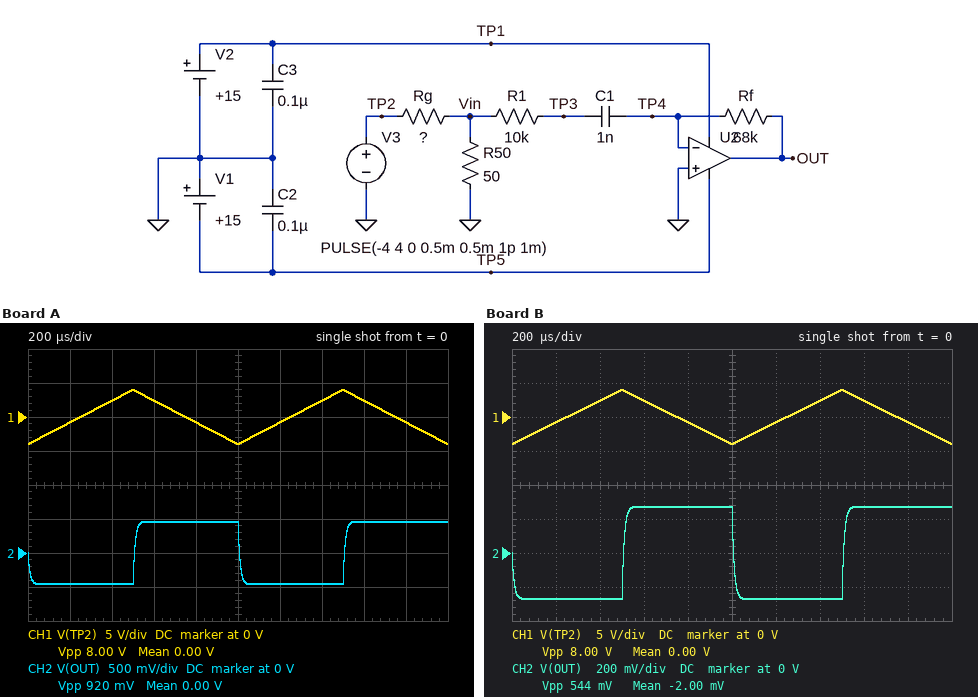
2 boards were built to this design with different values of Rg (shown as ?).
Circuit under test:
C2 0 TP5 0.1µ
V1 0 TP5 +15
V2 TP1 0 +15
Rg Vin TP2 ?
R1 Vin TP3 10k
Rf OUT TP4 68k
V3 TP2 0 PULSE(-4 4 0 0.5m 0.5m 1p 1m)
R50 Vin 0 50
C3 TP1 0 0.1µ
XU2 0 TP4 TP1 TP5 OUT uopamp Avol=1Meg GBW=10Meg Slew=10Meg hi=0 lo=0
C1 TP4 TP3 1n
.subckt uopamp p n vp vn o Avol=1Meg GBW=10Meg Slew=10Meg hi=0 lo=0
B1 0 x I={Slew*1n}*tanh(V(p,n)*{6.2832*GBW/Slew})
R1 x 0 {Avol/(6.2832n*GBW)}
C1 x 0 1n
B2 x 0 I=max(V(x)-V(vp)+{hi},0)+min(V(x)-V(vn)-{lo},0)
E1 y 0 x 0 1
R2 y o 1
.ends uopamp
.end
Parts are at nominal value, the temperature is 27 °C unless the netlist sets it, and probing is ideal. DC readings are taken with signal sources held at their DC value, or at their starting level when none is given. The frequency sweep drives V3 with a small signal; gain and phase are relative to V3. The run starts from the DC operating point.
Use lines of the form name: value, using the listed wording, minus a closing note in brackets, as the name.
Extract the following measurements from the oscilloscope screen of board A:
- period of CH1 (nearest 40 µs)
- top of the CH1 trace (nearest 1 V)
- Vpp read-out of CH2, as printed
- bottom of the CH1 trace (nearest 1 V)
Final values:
period of CH1: 1.00 ms
top of the CH1 trace: 4 V
Vpp read-out of CH2, as printed: 920 mV
bottom of the CH1 trace: -4 V
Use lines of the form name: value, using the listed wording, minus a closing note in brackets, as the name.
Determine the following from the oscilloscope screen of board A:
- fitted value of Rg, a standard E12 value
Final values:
fitted value of Rg, a standard E12 value: 68 Ω
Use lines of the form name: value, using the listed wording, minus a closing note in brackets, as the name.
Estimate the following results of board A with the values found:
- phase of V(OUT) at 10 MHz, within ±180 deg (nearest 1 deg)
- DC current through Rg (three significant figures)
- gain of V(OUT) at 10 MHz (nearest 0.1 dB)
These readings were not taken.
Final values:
phase of V(OUT) at 10 MHz, within ±180 deg: 97 deg
DC current through Rg: 33.9 mA
gain of V(OUT) at 10 MHz: -8.7 dB
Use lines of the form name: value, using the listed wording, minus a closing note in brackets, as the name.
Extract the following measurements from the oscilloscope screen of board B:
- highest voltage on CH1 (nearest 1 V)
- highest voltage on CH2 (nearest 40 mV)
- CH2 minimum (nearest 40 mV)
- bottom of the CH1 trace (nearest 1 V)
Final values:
highest voltage on CH1: 4 V
highest voltage on CH2: 280 mV
CH2 minimum: -280 mV
bottom of the CH1 trace: -4 V
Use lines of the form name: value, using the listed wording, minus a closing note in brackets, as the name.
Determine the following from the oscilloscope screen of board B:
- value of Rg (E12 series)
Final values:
value of Rg: 150 Ω
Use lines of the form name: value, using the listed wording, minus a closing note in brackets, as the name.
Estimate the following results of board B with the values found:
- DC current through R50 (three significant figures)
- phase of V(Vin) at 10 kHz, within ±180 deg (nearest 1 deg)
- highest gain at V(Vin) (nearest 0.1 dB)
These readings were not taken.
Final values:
DC current through R50: 20.0 mA
phase of V(Vin) at 10 kHz, within ±180 deg: 0 deg
highest gain at V(Vin): -12.0 dB
